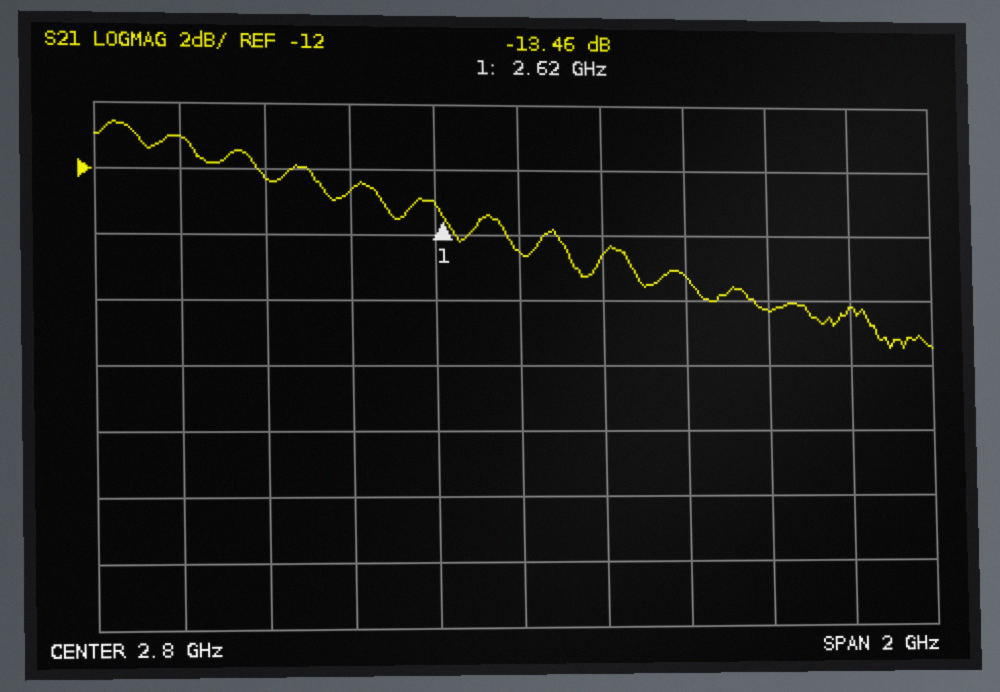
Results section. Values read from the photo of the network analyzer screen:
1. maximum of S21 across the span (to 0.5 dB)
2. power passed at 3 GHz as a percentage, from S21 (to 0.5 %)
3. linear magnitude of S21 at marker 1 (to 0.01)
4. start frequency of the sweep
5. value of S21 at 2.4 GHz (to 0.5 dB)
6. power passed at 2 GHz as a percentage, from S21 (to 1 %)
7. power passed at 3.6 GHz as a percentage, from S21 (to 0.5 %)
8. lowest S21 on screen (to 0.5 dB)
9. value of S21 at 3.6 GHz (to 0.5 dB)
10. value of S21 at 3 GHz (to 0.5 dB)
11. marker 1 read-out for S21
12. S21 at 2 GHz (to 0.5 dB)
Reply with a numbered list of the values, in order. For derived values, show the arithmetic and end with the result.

1. -10.5 dB
2. 10^(-14.5/10) ≈ 3.5 %
3. 10^(-13.46/20) ≈ 0.21
4. 1.8 GHz
5. -12.5 dB
6. 10^(-11/10) ≈ 8 %
7. 10^(-16/10) ≈ 2.5 %
8. -17.5 dB
9. -16.0 dB
10. -14.5 dB
11. -13.46 dB
12. -11.0 dB
